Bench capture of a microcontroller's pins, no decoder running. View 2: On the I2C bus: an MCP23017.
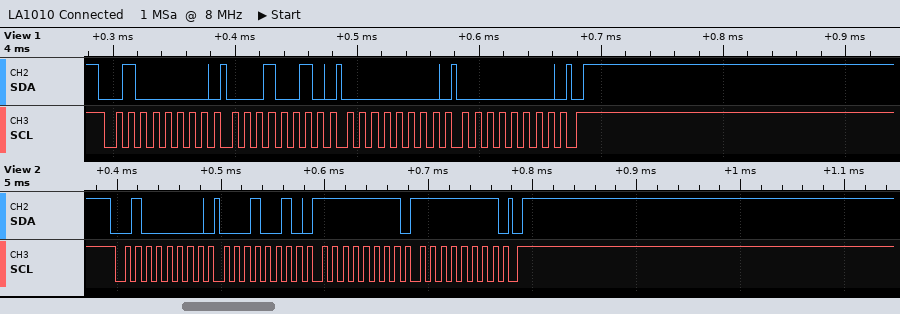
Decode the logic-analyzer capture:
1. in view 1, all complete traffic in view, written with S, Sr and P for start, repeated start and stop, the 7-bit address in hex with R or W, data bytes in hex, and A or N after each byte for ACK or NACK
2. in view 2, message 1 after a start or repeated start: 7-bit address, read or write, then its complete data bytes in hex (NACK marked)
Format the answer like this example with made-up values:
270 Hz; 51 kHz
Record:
S 20W A 12 A 00 A 00 A P; 0x20 write: 12 FF FF
